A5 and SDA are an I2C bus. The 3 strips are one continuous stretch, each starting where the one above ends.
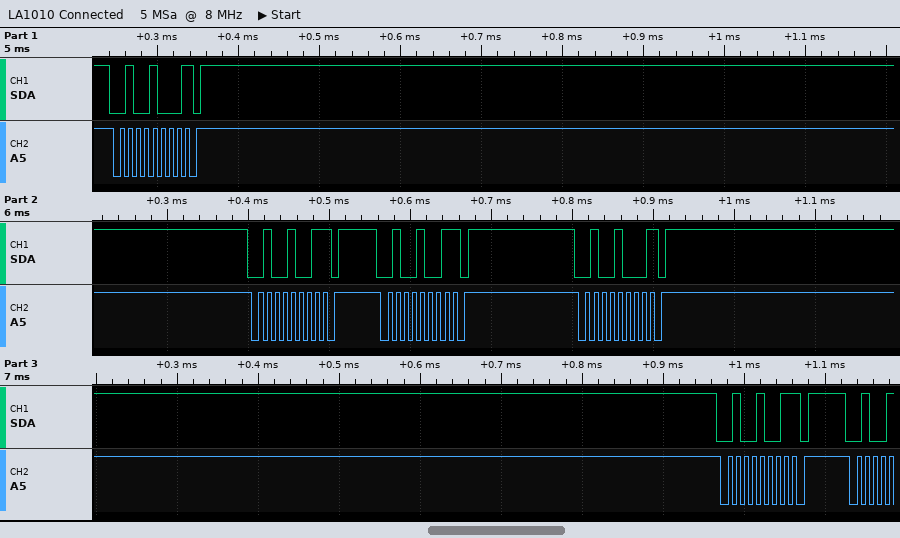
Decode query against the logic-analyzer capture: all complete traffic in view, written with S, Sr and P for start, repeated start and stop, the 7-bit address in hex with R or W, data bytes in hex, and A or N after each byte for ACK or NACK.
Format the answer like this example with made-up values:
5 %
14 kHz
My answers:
S 24W N P S 24R N P S 24R N P S 24W N P S 24R N P
